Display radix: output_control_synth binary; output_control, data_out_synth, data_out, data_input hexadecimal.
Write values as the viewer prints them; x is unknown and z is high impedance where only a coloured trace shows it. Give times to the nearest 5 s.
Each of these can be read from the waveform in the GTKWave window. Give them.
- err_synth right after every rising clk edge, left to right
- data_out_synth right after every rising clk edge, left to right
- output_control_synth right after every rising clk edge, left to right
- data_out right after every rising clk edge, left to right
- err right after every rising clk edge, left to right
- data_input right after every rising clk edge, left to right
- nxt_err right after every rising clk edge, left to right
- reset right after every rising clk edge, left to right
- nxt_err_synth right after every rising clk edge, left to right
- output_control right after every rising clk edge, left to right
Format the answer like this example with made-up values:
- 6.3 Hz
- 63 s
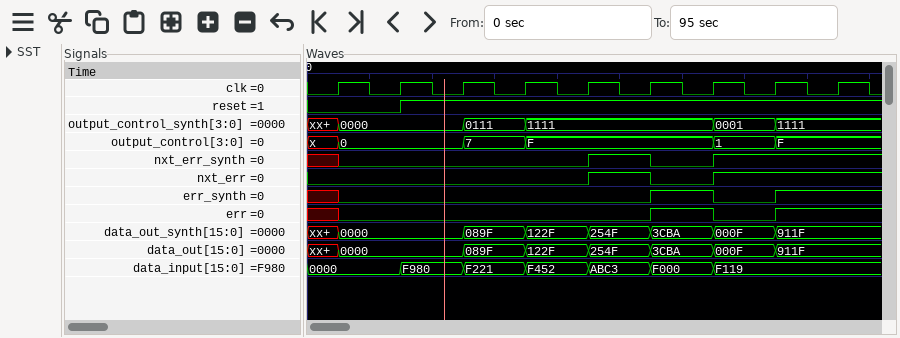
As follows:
- 0 0 0 0 0 1 0 1 1
- 0000, 0000, 089F, 122F, 254F, 3CBA, 000F, 911F, 911F
- 0000, 0000, 0111, 1111, 1111, 1111, 0001, 1111, 1111
- 0000, 0000, 089F, 122F, 254F, 3CBA, 000F, 911F, 911F
- 0 0 0 0 0 1 0 1 1
- 0000, F980, F221, F452, ABC3, F000, F119, F119, F119
- 0 0 0 0 1 0 1 1 1
- 0 1 1 1 1 1 1 1 1
- 0 0 0 0 1 0 1 1 1
- 0, 0, 7, F, F, F, 1, F, F
